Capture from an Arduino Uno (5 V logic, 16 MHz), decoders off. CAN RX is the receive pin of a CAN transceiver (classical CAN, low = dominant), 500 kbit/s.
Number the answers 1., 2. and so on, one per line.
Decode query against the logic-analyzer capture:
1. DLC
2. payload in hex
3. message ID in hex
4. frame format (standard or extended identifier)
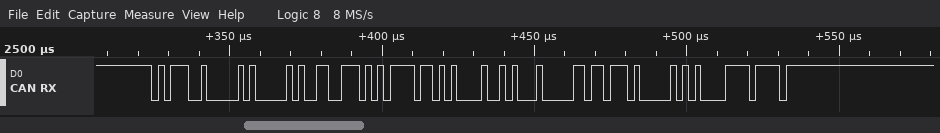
1. 8
2. 13 3A BD A8 4A 20 B7 40
3. 0x5C8
4. standard
